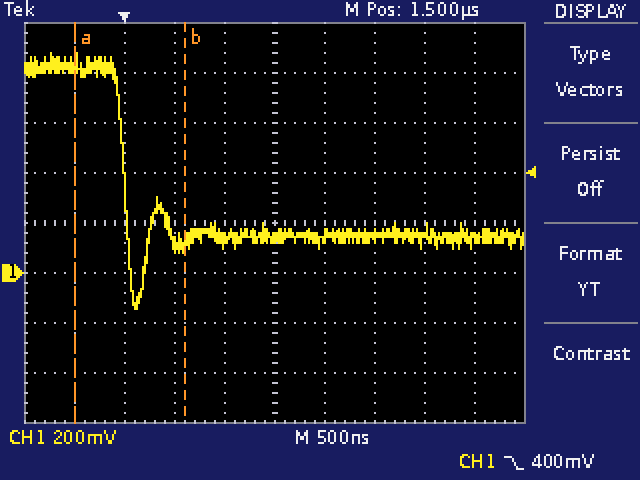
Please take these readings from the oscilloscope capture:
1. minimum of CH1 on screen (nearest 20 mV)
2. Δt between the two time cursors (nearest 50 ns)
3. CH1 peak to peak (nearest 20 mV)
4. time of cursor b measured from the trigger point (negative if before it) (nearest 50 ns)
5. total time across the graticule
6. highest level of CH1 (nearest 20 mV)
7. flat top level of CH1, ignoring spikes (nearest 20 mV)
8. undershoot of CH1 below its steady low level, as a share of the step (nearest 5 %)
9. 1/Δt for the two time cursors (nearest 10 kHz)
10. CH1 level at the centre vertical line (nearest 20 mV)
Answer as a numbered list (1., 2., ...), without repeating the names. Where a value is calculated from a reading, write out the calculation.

1. -140 mV
2. 1.10 µs
3. 880 mV − (-140 mV) = 1.02 V
4. +600 ns
5. 5 µs
6. 880 mV
7. 820 mV
8. 45 %
9. 1 / 1.10 µs ≈ 910 kHz
10. 140 mV
